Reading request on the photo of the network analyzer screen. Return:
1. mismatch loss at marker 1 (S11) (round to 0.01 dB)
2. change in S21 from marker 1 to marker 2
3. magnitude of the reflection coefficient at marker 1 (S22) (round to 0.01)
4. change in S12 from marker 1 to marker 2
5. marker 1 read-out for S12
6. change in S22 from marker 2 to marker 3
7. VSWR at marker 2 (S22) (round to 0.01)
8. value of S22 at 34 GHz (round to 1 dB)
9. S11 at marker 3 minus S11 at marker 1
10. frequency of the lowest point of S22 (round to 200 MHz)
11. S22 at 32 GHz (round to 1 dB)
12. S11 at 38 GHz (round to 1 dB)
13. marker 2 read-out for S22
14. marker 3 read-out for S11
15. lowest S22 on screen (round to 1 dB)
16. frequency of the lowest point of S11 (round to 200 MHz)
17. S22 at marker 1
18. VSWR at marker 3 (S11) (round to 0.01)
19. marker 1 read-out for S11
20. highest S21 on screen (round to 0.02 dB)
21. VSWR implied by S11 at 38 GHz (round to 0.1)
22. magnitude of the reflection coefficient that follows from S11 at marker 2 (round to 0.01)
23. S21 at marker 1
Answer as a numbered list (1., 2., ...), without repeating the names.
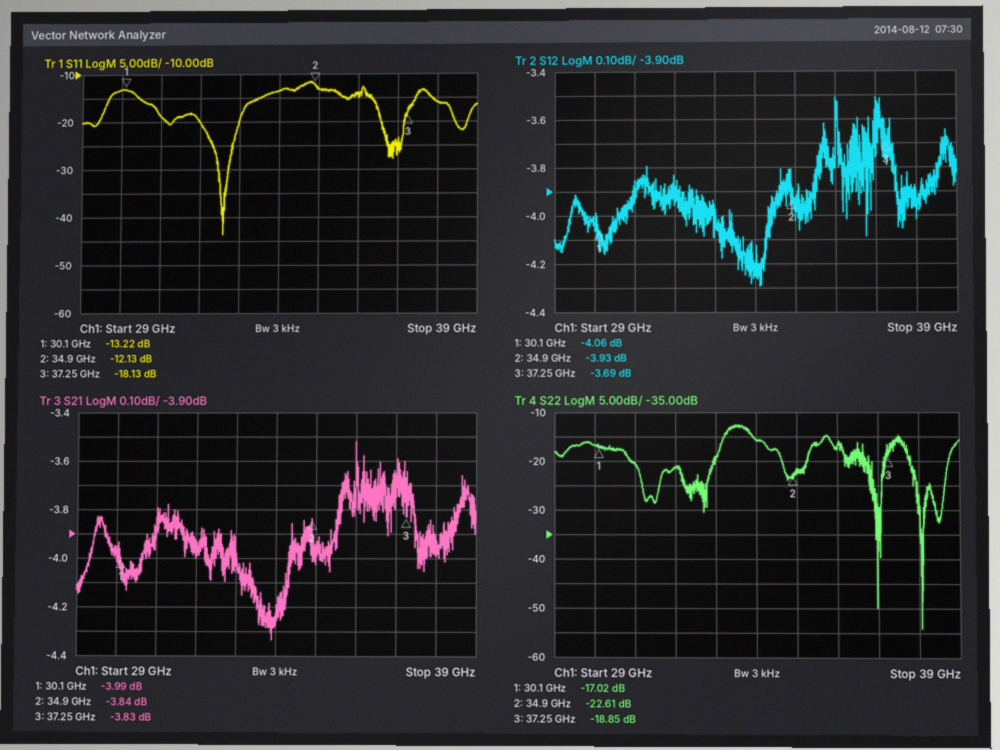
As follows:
1. 0.21 dB
2. 0.15 dB
3. 0.14
4. 0.13 dB
5. -4.06 dB
6. 3.76 dB
7. 1.16
8. -16 dB
9. -4.91 dB
10. 38.0 GHz
11. -21 dB
12. -16 dB
13. -22.61 dB
14. -18.13 dB
15. -54 dB
16. 32.6 GHz
17. -17.02 dB
18. 1.28
19. -13.22 dB
20. -3.52 dB
21. 1.4
22. 0.25
23. -3.99 dB
